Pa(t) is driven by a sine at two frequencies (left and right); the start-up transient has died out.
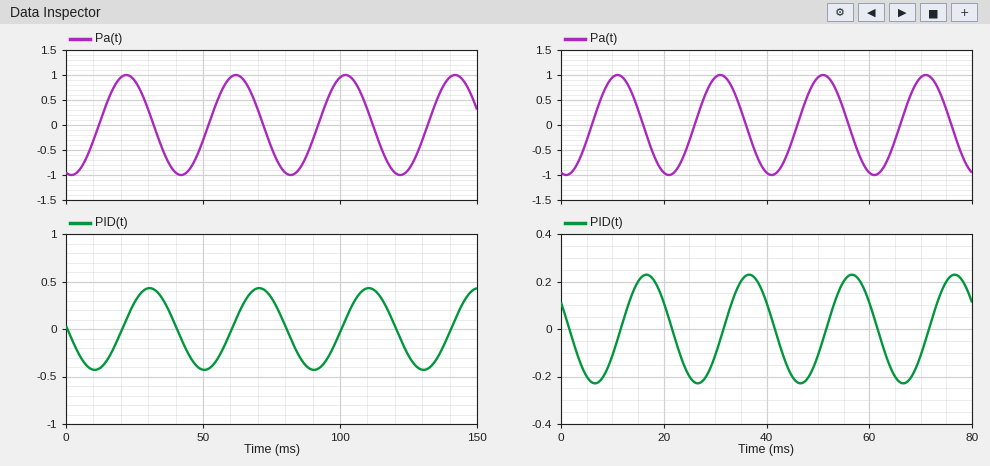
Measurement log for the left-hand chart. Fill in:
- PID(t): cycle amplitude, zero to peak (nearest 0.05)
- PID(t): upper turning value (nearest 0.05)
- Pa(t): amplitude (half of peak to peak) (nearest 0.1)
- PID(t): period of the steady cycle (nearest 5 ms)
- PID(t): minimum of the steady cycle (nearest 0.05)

0.45
0.45
1.0
40 ms
-0.45
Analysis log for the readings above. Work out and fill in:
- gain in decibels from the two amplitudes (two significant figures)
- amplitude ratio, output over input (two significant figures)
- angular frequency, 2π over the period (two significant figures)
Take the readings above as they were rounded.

-6.9 dB
0.45
0.16 rad/ms
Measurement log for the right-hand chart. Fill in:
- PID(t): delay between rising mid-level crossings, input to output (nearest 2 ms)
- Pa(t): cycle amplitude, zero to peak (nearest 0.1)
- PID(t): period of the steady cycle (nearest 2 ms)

6 ms
1.0
20 ms
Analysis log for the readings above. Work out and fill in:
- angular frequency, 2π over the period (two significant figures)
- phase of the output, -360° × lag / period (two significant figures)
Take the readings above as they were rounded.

0.31 rad/ms
-110°
